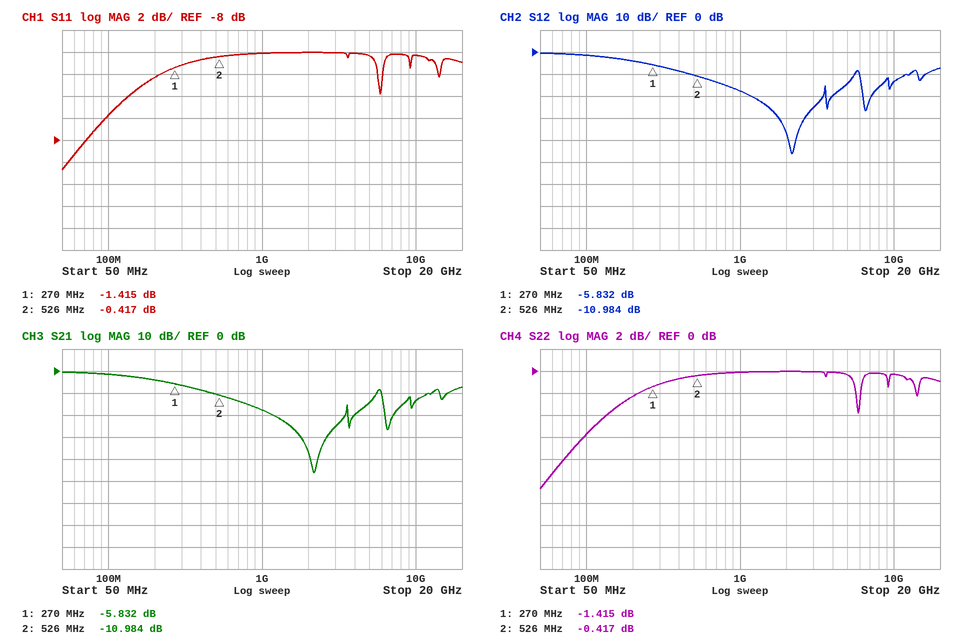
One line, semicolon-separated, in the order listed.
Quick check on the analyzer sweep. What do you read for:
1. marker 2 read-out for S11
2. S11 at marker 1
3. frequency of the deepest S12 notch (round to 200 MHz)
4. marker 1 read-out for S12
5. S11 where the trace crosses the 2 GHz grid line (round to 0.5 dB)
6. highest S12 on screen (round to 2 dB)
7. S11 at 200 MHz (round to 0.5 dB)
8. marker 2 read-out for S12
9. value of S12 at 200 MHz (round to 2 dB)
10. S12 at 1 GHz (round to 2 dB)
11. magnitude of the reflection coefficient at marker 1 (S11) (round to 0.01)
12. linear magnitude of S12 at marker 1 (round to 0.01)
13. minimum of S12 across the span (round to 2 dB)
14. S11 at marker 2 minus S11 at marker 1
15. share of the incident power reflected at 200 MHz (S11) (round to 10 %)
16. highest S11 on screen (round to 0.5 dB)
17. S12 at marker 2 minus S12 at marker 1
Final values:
-0.417 dB; -1.415 dB; 2.2 GHz; -5.832 dB; 0.0 dB; 0 dB; -2.5 dB; -10.984 dB; -4 dB; -18 dB; 0.85; 0.51; -46 dB; 0.998 dB; 60 %; 0.0 dB; -5.152 dB
